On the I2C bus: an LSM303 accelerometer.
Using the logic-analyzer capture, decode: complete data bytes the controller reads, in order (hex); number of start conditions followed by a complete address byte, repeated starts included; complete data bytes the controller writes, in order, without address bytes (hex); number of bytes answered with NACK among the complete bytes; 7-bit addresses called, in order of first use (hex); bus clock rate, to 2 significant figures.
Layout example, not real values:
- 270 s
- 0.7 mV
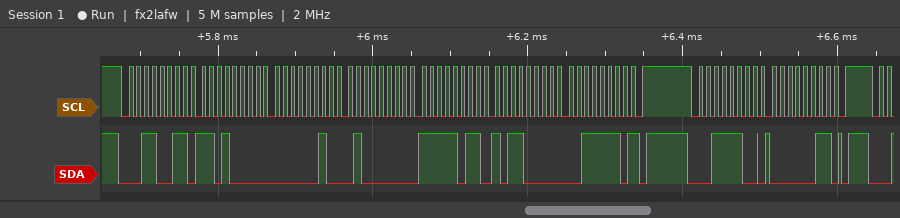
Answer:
- D0 02 40 FB B0 3E
- 2
- 03
- 1
- 0x19 0x1E
- 100 kHz
